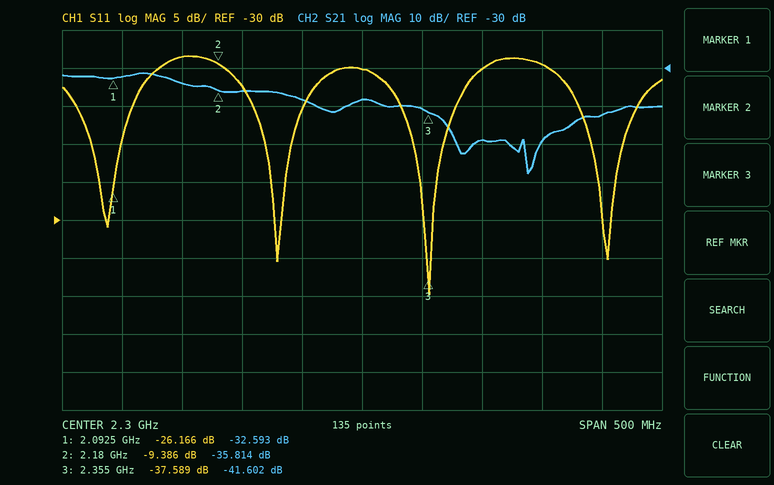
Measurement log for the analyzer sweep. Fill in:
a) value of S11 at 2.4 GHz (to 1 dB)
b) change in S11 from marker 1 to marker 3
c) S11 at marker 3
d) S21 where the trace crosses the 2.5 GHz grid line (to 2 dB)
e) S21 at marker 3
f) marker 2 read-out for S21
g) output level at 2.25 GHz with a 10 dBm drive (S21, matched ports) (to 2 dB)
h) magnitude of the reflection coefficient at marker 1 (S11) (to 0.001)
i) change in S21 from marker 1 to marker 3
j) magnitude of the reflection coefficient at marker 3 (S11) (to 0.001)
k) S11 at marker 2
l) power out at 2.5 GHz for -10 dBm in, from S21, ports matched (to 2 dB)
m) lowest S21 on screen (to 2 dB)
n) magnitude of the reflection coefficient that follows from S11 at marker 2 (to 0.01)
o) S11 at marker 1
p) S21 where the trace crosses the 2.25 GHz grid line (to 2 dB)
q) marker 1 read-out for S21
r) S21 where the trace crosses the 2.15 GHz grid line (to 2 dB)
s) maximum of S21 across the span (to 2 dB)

-10 dB
-11.423 dB
-37.589 dB
-42 dB
-41.602 dB
-35.814 dB
-28 dBm
0.049
-9.009 dB
0.013
-9.386 dB
-52 dBm
-58 dB
0.34
-26.166 dB
-38 dB
-32.593 dB
-34 dB
-32 dB
